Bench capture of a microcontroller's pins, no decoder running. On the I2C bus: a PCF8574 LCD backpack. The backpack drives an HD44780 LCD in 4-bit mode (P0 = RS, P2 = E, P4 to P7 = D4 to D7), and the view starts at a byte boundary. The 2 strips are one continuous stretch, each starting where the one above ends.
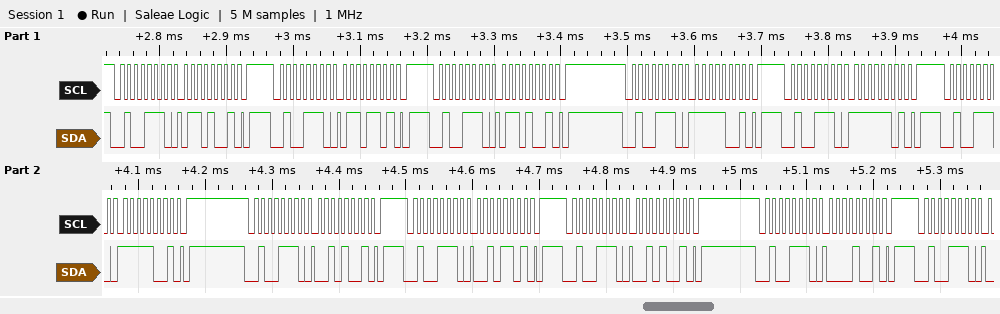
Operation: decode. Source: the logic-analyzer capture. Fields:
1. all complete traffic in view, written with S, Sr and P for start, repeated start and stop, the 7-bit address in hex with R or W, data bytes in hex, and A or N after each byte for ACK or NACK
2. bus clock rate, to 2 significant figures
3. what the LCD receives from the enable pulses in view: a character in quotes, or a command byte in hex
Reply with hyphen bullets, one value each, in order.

- S 27W A 69 A P S 27W A 6D A P S 27W A 69 A P S 27W A F9 A P S 27W A FD A P S 27W A F9 A P S 27W A 29 A P S 27W A 2D A P S 27W A 29 A P S 27W A 09 A P S 27W A
- 100 kHz
- 'o'
